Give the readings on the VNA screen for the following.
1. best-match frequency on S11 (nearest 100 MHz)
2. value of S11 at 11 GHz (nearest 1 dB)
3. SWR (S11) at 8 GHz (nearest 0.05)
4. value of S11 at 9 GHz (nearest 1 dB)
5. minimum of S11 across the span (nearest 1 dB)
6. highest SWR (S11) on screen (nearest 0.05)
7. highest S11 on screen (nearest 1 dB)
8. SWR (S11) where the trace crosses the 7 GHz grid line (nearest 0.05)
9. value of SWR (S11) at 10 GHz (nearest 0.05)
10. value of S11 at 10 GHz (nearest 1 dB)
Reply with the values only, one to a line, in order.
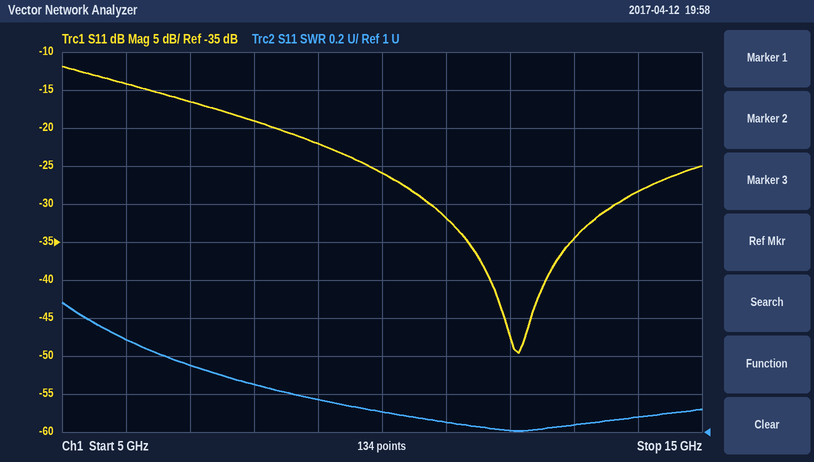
12.1 GHz
-32 dB
1.25
-22 dB
-50 dB
1.70
-12 dB
1.35
1.10
-26 dB
